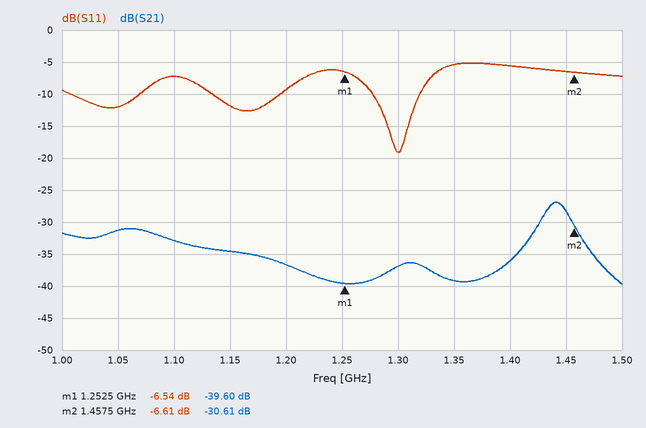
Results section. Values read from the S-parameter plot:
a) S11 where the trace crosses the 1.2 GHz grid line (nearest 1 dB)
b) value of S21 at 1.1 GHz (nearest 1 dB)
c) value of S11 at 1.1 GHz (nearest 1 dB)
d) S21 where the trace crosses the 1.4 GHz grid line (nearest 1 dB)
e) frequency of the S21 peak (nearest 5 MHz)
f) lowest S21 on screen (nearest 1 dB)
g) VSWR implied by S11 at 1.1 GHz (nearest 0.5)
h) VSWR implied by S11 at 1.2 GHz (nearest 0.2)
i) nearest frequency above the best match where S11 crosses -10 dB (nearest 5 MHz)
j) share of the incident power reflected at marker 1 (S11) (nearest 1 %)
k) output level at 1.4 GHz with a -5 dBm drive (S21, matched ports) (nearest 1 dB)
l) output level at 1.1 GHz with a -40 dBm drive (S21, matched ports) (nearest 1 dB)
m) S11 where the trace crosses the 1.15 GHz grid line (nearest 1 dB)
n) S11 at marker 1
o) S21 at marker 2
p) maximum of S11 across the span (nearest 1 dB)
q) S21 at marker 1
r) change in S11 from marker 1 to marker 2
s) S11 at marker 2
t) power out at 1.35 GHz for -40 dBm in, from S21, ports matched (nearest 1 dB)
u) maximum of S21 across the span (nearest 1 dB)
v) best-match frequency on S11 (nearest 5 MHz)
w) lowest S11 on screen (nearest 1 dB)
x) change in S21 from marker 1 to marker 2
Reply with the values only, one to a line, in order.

-9 dB
-33 dB
-7 dB
-36 dB
1.440 GHz
-40 dB
2.5
2.0
1.320 GHz
22 %
-41 dBm
-73 dBm
-12 dB
-6.54 dB
-30.61 dB
-5 dB
-39.60 dB
-0.07 dB
-6.61 dB
-79 dBm
-27 dB
1.300 GHz
-19 dB
8.99 dB
